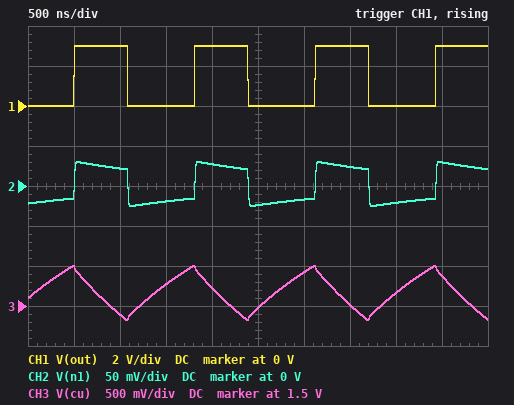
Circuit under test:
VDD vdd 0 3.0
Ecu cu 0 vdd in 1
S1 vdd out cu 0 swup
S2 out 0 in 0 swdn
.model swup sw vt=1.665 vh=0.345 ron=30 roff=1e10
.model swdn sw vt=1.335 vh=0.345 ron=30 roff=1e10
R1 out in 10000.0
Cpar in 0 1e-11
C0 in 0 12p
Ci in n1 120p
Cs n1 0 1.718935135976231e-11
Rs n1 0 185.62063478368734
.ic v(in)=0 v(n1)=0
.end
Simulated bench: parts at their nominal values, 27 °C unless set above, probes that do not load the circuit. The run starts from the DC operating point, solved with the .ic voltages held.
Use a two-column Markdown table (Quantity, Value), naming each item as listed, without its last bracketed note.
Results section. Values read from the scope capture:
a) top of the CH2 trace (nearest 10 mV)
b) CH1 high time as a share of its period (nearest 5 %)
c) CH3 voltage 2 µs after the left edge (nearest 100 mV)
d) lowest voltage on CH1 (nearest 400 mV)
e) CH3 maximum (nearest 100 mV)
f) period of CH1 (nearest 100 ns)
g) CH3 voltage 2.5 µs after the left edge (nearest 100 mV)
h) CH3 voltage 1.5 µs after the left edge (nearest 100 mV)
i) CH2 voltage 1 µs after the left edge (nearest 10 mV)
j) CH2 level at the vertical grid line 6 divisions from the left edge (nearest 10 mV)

| Quantity | Value |
|---|---|
| top of the CH2 trace | 30 mV |
| CH1 high time as a share of its period | 45 % |
| CH3 voltage 2 µs after the left edge | 1.7 V |
| lowest voltage on CH1 | 0 V |
| CH3 maximum | 2.0 V |
| period of CH1 | 1.3 µs |
| CH3 voltage 2.5 µs after the left edge | 1.5 V |
| CH3 voltage 1.5 µs after the left edge | 1.8 V |
| CH2 voltage 1 µs after the left edge | 20 mV |
| CH2 level at the vertical grid line 6 divisions from the left edge | -20 mV |
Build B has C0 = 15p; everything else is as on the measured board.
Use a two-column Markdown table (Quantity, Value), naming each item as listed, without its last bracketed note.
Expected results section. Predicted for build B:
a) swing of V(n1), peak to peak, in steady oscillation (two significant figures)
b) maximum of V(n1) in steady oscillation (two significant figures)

| Quantity | Value |
|---|---|
| swing of V(n1), peak to peak, in steady oscillation | 54 mV |
| maximum of V(n1) in steady oscillation | 29 mV |
